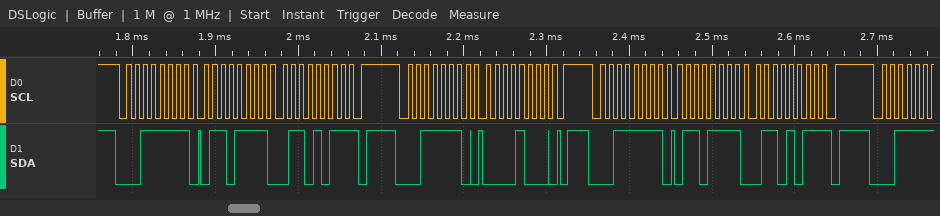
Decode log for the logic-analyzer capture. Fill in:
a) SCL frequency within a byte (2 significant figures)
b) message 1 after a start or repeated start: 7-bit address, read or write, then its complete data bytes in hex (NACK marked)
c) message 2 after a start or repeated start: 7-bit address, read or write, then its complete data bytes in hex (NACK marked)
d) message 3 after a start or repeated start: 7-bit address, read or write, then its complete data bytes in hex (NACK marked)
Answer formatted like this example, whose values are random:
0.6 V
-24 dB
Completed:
100 kHz
0x1F read: 6F 6B NACK
0x1F write: 08
0x1F read: 6F 6B NACK
